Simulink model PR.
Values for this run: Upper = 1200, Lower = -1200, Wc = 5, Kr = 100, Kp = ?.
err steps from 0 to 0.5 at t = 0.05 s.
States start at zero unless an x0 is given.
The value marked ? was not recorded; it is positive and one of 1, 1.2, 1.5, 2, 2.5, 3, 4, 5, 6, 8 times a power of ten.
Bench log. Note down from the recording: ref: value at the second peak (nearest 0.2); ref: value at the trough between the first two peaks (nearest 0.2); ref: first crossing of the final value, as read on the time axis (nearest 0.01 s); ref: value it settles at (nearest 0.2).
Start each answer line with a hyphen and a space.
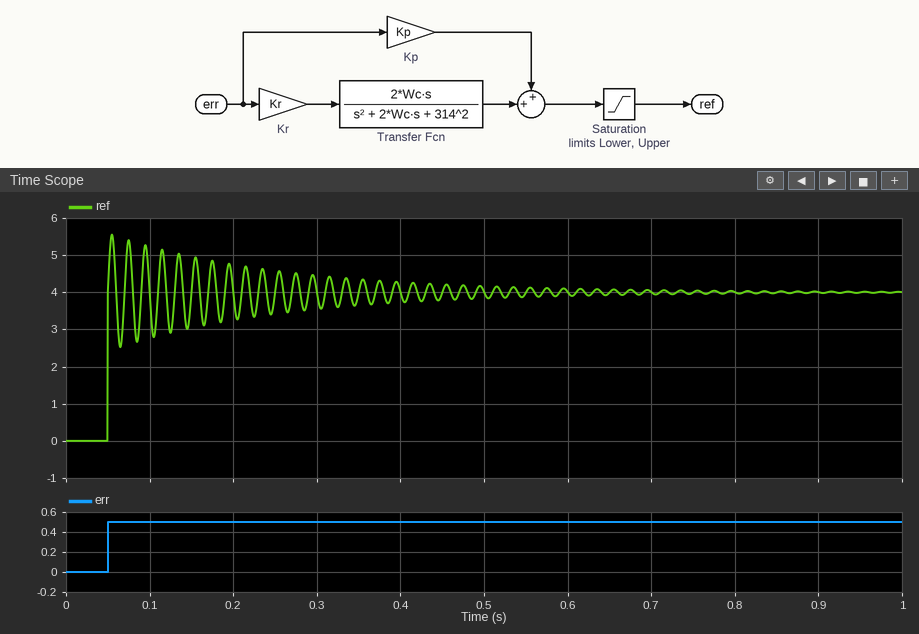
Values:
- 5.4
- 2.6
- 0.05 s
- 4.0
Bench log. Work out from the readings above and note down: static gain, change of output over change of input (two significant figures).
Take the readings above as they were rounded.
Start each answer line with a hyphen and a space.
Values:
- 8.0
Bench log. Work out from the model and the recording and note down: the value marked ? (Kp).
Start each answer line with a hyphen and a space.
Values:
- 8
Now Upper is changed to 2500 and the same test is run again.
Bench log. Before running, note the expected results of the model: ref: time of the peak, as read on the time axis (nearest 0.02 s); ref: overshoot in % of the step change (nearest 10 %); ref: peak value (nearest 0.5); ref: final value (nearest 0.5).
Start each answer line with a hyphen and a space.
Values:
- 0.06 s
- 40 %
- 5.5
- 4.0
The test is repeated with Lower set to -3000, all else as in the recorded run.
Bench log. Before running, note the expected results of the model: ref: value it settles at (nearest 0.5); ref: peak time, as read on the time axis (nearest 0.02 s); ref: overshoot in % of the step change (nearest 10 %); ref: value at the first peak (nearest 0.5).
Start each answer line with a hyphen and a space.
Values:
- 4.0
- 0.06 s
- 40 %
- 5.5
